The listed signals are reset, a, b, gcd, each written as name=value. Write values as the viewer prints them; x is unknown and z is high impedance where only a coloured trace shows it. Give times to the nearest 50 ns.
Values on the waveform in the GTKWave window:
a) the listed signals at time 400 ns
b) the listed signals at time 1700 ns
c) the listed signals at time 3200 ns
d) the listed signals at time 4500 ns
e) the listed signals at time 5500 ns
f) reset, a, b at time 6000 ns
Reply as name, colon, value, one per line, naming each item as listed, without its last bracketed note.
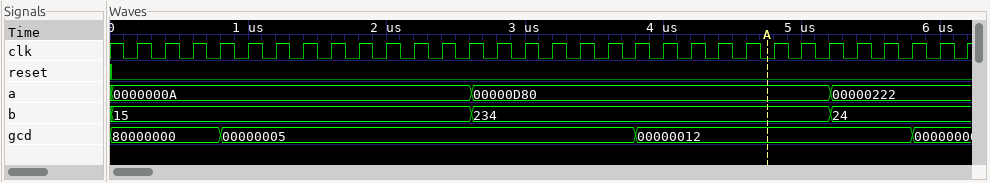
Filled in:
the listed signals at time 400 ns: reset=0, a=0000000A, b=15, gcd=80000000
the listed signals at time 1700 ns: reset=0, a=0000000A, b=15, gcd=00000005
the listed signals at time 3200 ns: reset=0, a=00000D80, b=234, gcd=00000005
the listed signals at time 4500 ns: reset=0, a=00000D80, b=234, gcd=00000012
the listed signals at time 5500 ns: reset=0, a=00000222, b=24, gcd=00000012
reset, a, b at time 6000 ns: reset=0, a=00000222, b=24
